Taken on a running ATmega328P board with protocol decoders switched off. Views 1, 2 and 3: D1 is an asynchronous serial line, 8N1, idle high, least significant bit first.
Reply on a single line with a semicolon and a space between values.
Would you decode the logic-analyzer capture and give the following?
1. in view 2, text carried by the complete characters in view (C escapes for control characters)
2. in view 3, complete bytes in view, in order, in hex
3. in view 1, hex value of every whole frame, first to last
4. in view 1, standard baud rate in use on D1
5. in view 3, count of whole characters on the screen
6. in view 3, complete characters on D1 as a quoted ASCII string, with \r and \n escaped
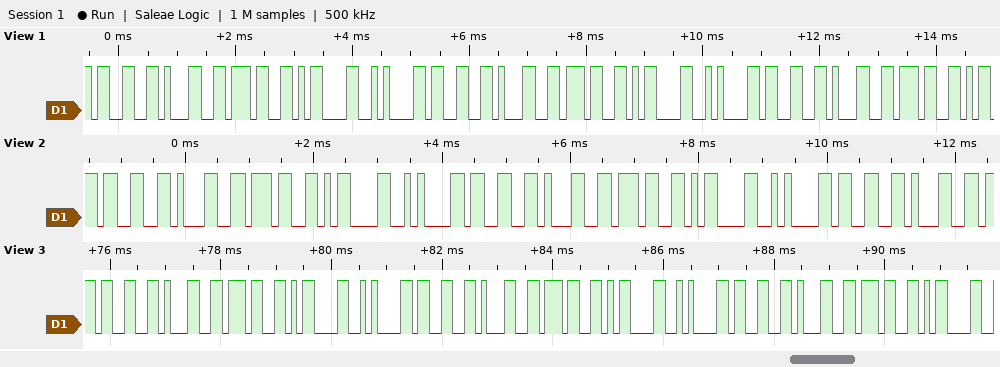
"317\r\n317\r\n31"; 33 31 37 0D 0A 33 31 37 0D 0A 33 31 37 0D; 0x33 0x31 0x37 0x0D 0x0A 0x33 0x31 0x37 0x0D 0x0A 0x33 0x31 0x37; 9600 baud; 14; "317\r\n317\r\n317\r"
